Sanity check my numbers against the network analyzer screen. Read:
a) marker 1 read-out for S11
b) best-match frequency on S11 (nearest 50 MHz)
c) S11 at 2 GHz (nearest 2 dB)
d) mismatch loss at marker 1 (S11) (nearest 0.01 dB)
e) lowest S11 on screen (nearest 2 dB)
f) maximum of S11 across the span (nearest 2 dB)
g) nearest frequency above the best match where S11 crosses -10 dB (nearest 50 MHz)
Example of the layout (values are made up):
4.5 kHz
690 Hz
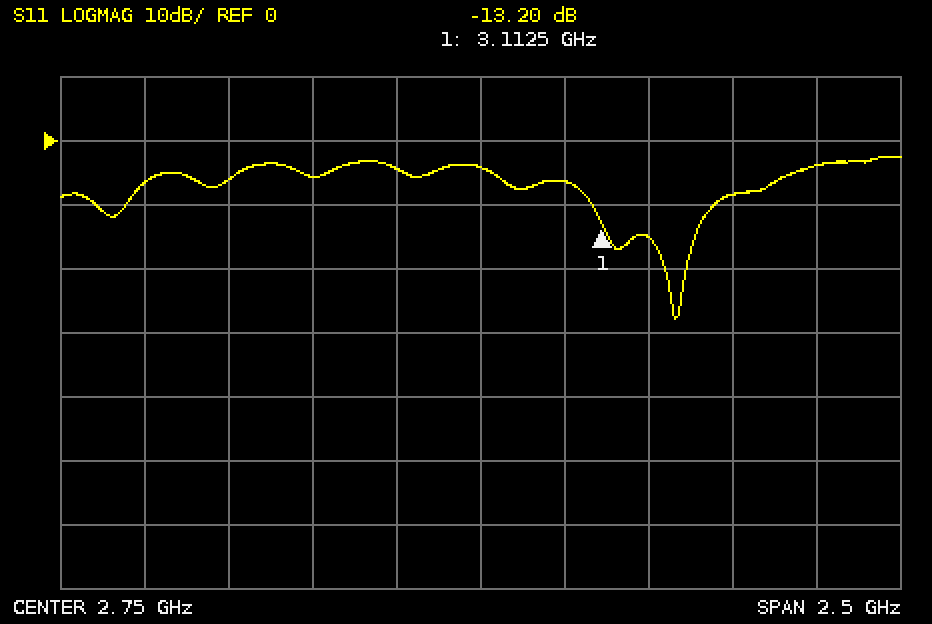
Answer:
-13.20 dB
3.35 GHz
-6 dB
0.21 dB
-28 dB
-2 dB
3.45 GHz
